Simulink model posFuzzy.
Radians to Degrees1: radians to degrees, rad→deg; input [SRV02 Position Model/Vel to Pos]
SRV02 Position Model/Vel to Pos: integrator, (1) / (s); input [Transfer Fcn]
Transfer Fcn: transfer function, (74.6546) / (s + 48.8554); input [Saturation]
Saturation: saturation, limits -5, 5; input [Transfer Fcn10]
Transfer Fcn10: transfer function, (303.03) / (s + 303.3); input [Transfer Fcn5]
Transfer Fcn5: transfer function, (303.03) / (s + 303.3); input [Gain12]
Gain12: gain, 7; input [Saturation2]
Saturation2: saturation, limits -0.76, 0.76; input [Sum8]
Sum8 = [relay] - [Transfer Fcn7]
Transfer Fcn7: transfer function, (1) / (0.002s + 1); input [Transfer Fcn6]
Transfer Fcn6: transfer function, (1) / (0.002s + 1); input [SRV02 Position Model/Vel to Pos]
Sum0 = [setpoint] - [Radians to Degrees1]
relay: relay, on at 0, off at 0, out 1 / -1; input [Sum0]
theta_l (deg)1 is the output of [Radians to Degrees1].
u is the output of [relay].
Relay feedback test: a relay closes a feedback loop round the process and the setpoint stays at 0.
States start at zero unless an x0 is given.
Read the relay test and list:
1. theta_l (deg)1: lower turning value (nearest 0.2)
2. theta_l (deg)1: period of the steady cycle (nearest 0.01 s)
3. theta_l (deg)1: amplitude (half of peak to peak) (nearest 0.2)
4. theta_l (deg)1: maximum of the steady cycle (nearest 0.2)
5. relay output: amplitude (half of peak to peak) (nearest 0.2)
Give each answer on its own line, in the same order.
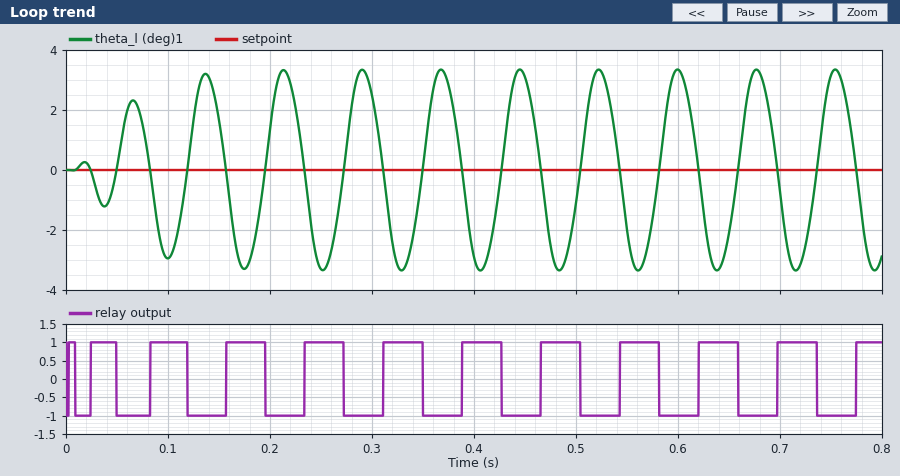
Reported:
-3.4
0.08 s
3.4
3.4
1.0
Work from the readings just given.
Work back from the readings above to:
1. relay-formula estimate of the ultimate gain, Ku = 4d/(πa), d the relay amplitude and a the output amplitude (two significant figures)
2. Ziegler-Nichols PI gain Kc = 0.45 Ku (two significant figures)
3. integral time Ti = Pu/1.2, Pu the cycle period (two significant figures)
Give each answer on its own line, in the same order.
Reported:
0.37
0.17
0.067 s
